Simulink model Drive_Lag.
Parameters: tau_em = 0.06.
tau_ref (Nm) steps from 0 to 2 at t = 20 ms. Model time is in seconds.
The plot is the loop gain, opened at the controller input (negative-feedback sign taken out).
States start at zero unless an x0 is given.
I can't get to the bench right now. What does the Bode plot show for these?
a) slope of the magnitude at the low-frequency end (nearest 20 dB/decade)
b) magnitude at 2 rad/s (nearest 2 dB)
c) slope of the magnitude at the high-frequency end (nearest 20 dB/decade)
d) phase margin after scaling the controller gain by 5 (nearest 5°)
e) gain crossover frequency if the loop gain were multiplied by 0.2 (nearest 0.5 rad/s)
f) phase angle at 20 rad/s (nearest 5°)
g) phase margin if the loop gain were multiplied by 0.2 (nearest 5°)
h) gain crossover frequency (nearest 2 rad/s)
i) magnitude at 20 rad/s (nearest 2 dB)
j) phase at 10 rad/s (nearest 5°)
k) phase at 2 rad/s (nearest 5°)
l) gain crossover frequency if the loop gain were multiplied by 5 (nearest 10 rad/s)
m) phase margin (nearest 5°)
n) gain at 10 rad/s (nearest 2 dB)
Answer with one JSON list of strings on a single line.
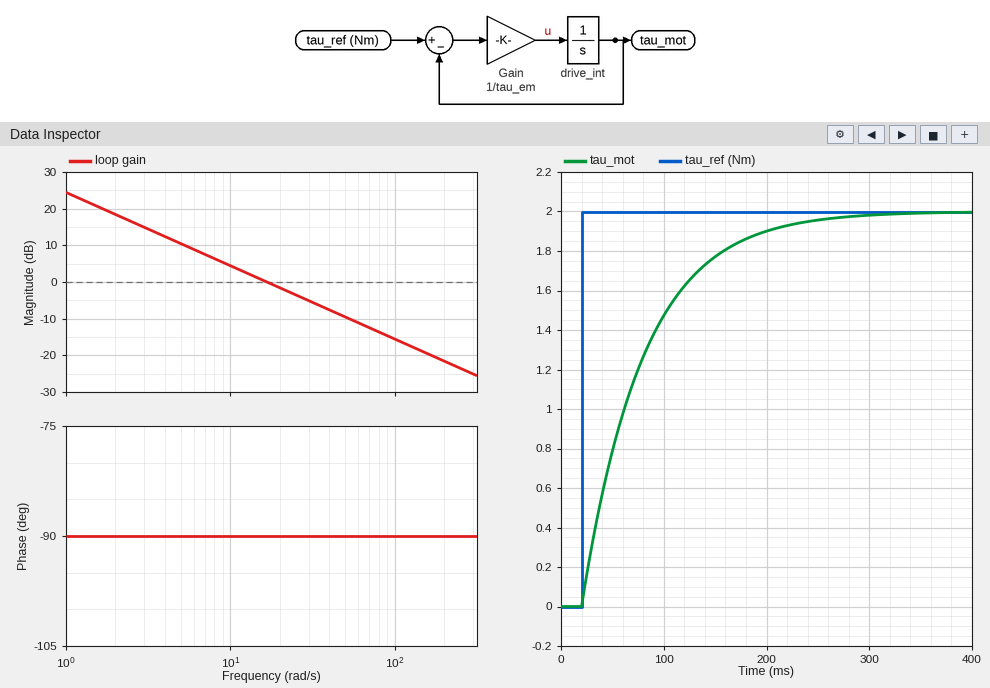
["-20 dB/decade", "18 dB", "-20 dB/decade", "90°", "3.5 rad/s", "-90°", "90°", "16 rad/s", "-2 dB", "-90°", "-90°", "80 rad/s", "90°", "4 dB"]
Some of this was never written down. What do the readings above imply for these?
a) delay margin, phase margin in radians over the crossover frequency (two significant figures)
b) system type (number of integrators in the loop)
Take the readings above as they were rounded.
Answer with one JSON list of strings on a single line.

["0.098 s", "1"]
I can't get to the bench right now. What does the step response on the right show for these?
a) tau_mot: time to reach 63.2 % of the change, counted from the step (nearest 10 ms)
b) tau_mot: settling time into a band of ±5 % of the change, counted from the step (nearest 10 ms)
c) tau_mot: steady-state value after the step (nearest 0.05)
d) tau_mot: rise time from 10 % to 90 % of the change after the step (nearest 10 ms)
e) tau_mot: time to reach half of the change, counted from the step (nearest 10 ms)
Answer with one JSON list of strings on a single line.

["60 ms", "180 ms", "2.00", "130 ms", "40 ms"]
